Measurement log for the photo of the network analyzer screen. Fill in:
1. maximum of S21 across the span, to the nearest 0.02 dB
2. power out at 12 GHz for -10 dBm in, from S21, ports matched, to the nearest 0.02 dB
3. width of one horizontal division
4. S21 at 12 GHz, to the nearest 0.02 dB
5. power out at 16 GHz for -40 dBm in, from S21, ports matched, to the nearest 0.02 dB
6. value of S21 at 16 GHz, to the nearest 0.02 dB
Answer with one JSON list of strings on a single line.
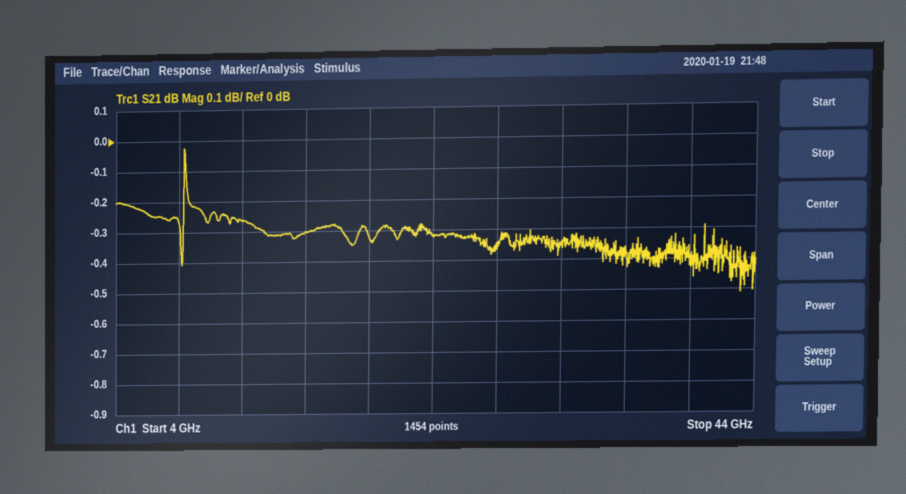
["-0.02 dB", "-10.26 dBm", "4 GHz", "-0.26 dB", "-40.30 dBm", "-0.30 dB"]
